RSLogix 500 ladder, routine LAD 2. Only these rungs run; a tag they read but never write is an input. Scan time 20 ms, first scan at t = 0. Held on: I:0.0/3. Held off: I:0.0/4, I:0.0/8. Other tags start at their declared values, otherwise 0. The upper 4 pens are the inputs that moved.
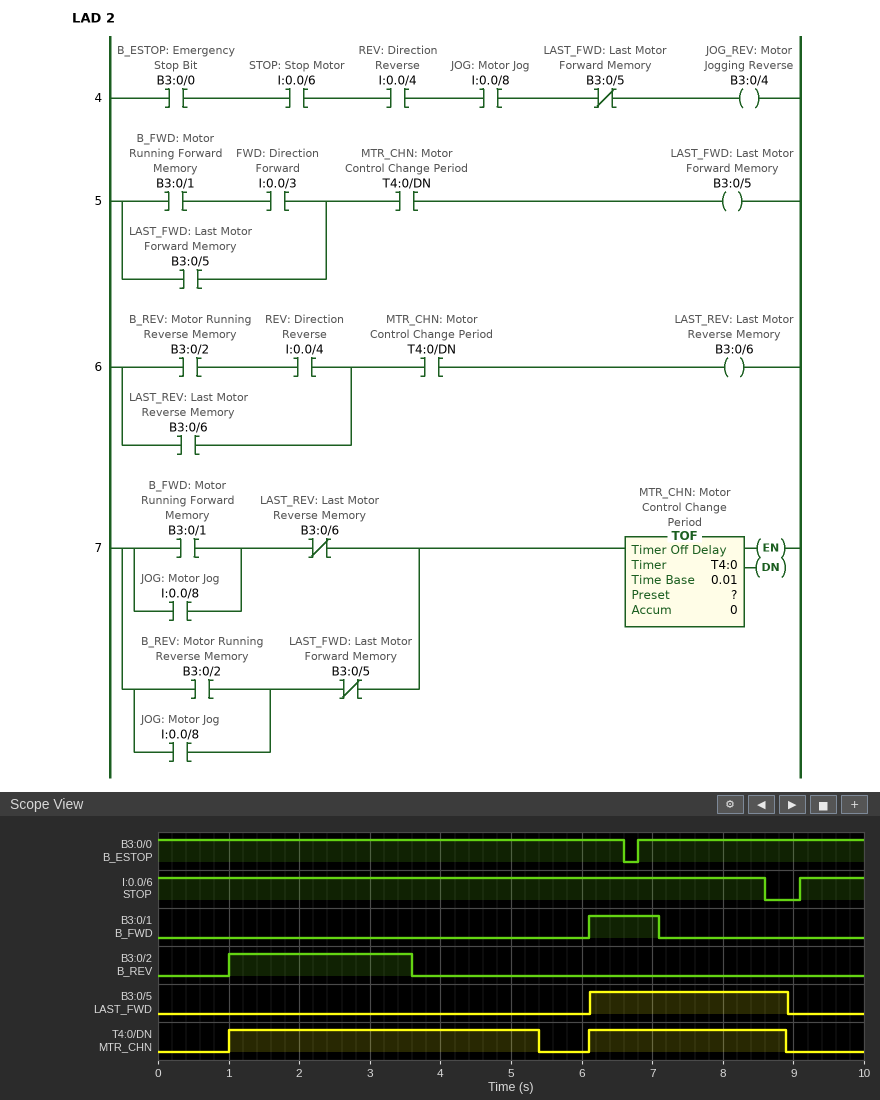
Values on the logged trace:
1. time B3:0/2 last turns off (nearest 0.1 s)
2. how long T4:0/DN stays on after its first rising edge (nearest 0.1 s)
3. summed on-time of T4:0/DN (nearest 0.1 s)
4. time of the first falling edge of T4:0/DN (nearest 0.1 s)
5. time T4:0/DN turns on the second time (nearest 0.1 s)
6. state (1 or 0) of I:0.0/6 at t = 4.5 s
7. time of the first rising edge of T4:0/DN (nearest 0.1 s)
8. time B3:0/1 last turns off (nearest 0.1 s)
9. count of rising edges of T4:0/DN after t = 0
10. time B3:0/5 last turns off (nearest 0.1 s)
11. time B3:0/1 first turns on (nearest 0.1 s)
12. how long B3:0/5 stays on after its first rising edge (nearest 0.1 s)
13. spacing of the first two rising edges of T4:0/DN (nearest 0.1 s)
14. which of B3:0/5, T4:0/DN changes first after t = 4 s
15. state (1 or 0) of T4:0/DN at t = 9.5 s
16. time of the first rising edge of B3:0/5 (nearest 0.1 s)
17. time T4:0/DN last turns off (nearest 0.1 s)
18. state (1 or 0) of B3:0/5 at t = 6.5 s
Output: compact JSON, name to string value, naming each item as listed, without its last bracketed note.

{"time B3:0/2 last turns off": "3.6 s", "how long T4:0/DN stays on after its first rising edge": "4.4 s", "summed on-time of T4:0/DN": "7.2 s", "time of the first falling edge of T4:0/DN": "5.4 s", "time T4:0/DN turns on the second time": "6.1 s", "state (1 or 0) of I:0.0/6 at t = 4.5 s": "1", "time of the first rising edge of T4:0/DN": "1.0 s", "time B3:0/1 last turns off": "7.1 s", "count of rising edges of T4:0/DN after t = 0": "2", "time B3:0/5 last turns off": "8.9 s", "time B3:0/1 first turns on": "6.1 s", "how long B3:0/5 stays on after its first rising edge": "2.8 s", "spacing of the first two rising edges of T4:0/DN": "5.1 s", "which of B3:0/5, T4:0/DN changes first after t = 4 s": "T4:0/DN", "state (1 or 0) of T4:0/DN at t = 9.5 s": "0", "time of the first rising edge of B3:0/5": "6.1 s", "time T4:0/DN last turns off": "8.9 s", "state (1 or 0) of B3:0/5 at t = 6.5 s": "1"}
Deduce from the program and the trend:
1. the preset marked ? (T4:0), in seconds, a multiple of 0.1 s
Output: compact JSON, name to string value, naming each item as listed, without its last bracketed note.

{"the preset marked ? (T4:0), in seconds, a multiple of 0.1 s": "1.8 s"}
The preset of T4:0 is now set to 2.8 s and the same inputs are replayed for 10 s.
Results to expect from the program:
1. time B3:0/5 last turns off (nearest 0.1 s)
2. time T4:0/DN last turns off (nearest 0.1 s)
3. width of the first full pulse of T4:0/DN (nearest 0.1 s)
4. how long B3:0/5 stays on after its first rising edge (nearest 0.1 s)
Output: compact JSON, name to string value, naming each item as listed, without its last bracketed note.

{"time B3:0/5 last turns off": "9.9 s", "time T4:0/DN last turns off": "9.9 s", "width of the first full pulse of T4:0/DN": "8.9 s", "how long B3:0/5 stays on after its first rising edge": "3.8 s"}
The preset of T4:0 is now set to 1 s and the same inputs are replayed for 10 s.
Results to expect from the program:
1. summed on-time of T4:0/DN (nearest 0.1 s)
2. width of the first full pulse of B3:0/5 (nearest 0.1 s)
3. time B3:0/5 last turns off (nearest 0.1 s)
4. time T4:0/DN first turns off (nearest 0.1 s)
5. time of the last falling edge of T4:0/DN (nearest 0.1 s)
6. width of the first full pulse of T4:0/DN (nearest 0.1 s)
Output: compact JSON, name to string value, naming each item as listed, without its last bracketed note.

{"summed on-time of T4:0/DN": "5.6 s", "width of the first full pulse of B3:0/5": "2.0 s", "time B3:0/5 last turns off": "8.1 s", "time T4:0/DN first turns off": "4.6 s", "time of the last falling edge of T4:0/DN": "8.1 s", "width of the first full pulse of T4:0/DN": "3.6 s"}
